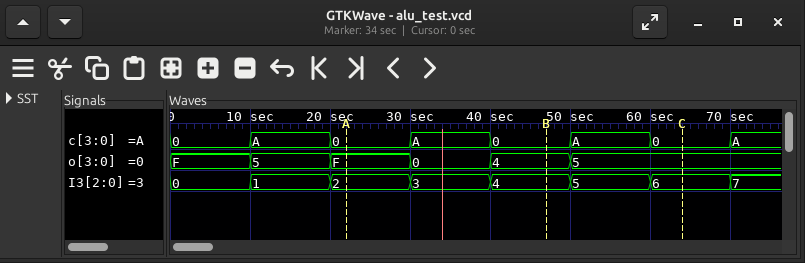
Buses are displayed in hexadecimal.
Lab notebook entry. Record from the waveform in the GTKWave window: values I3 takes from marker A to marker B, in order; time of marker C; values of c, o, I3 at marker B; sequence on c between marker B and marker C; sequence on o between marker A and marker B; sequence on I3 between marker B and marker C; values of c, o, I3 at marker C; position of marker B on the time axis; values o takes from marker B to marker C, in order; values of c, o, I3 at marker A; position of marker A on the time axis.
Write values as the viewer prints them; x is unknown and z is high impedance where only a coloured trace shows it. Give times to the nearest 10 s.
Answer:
2, 3, 4
60 s
c=0, o=4, I3=4
0, A, 0
F, 0, 4
4, 5, 6
c=0, o=5, I3=6
50 s
4, 5
c=0, o=F, I3=2
20 s
